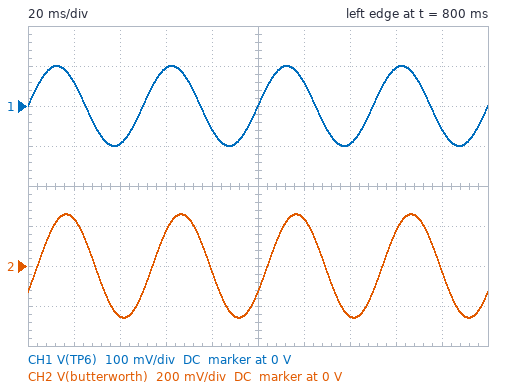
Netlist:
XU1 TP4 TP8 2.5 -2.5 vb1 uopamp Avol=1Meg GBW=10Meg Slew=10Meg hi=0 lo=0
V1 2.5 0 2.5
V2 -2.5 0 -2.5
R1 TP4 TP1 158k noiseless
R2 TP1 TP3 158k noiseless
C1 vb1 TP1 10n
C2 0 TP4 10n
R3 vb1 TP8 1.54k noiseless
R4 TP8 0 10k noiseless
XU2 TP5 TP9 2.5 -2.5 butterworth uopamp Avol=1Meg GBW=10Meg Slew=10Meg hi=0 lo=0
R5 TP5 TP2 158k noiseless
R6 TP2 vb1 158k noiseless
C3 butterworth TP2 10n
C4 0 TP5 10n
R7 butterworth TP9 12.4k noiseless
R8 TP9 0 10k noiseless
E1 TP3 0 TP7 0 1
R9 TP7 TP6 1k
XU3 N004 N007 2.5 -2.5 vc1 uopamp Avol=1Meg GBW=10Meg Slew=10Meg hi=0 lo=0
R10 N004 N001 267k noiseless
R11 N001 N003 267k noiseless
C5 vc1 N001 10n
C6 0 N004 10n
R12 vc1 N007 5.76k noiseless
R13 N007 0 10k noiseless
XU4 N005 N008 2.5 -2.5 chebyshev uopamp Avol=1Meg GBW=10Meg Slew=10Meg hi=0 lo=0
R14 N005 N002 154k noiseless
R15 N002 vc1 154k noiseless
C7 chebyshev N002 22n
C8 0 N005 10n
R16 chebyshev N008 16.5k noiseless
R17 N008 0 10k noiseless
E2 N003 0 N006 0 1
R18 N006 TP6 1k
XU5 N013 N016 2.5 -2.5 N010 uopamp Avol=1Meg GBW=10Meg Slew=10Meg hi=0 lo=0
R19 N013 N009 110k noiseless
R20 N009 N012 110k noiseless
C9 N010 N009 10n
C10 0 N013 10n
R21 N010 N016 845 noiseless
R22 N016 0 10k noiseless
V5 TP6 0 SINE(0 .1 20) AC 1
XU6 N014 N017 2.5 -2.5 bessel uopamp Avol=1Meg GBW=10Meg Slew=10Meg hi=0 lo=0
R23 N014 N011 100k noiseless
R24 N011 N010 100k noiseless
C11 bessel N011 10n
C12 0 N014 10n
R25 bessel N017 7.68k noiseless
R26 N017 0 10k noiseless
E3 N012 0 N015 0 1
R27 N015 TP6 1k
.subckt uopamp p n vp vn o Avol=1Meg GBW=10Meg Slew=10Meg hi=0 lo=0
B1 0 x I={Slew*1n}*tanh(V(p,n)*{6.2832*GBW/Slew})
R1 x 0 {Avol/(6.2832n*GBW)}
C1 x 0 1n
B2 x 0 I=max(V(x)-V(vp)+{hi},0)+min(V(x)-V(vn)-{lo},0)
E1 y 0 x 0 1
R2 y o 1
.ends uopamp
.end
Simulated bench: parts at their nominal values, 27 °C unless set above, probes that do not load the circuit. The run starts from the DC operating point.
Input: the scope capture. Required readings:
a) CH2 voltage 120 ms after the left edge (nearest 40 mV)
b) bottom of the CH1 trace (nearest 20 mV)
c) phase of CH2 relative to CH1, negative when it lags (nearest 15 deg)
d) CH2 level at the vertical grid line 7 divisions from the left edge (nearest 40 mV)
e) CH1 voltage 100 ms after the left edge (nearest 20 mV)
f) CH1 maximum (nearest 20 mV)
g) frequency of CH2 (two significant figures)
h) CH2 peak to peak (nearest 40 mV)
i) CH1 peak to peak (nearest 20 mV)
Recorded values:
240 mV
-100 mV
-30 deg
-240 mV
0 V
100 mV
20 Hz
520 mV
200 mV
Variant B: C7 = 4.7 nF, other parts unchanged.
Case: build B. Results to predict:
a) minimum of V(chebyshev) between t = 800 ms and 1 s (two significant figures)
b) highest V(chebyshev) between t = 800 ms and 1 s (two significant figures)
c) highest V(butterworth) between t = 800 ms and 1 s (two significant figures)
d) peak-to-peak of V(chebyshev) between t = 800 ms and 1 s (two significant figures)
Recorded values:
-410 mV
410 mV
260 mV
820 mV
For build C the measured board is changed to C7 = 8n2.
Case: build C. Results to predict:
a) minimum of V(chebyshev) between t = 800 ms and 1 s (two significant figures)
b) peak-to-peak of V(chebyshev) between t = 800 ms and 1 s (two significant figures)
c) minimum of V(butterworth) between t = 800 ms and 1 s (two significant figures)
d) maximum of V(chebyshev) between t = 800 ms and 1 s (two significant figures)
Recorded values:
-420 mV
850 mV
-260 mV
420 mV
